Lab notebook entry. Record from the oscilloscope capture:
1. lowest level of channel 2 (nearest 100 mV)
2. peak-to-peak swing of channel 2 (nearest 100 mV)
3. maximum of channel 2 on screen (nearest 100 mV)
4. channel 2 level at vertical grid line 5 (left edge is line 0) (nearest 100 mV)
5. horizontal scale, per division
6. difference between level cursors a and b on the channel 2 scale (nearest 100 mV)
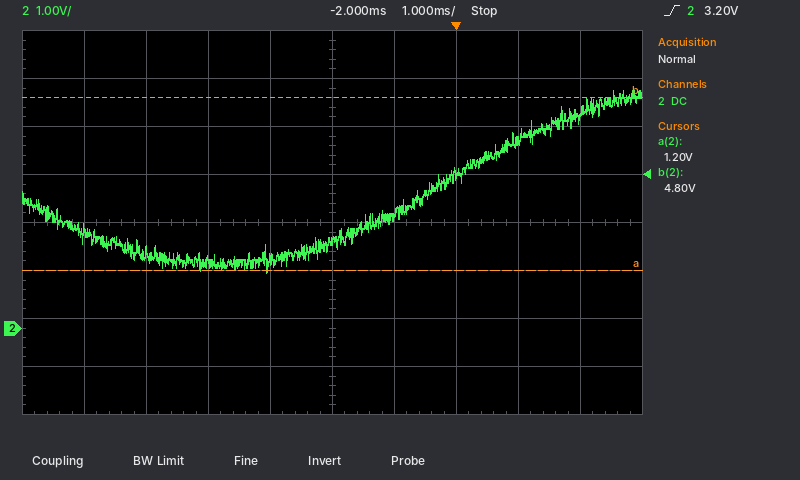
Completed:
1.2 V
3.8 V
5.0 V
1.8 V
1 ms
3.6 V
